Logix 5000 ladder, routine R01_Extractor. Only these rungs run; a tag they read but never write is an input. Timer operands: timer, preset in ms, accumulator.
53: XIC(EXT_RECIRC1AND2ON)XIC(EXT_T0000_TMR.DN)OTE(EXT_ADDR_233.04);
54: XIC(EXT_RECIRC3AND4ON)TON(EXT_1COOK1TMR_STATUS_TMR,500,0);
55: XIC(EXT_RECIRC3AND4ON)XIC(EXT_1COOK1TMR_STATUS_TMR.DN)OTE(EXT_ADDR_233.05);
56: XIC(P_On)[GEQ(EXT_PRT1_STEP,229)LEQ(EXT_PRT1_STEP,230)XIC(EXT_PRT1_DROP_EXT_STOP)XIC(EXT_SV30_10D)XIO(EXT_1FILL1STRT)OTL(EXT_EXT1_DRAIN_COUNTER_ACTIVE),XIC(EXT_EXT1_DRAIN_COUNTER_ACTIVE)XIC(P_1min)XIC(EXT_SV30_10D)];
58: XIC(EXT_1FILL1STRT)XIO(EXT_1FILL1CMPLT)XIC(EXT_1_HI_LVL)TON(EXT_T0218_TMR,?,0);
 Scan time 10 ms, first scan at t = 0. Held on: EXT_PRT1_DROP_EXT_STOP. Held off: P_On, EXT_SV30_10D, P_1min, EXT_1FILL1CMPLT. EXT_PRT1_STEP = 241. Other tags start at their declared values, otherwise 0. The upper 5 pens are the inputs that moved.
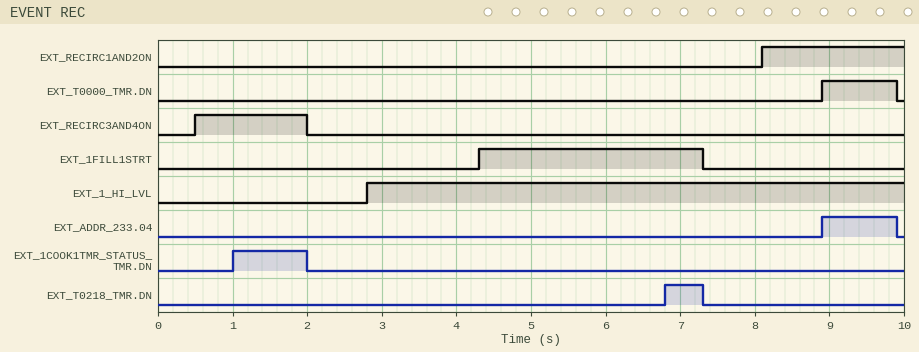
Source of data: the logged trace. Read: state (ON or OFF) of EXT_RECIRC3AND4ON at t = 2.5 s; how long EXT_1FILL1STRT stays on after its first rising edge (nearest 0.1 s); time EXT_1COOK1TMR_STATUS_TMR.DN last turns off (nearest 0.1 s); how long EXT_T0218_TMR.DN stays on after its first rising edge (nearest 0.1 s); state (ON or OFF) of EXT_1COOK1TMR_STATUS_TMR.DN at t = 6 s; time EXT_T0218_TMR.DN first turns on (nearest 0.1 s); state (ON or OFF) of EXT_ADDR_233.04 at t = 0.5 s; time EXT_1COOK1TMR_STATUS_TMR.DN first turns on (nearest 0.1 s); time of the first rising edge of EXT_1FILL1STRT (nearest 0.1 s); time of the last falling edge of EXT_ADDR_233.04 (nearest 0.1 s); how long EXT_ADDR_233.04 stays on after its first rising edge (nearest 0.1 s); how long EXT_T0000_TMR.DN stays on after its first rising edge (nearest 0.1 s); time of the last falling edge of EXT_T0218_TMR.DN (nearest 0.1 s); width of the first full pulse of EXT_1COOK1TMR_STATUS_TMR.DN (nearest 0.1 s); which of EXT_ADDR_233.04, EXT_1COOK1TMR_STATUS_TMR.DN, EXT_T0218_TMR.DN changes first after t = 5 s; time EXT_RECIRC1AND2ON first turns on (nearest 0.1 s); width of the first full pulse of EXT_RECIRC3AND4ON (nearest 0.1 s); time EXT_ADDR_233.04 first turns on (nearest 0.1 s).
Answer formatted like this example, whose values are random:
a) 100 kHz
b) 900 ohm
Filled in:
a) OFF
b) 3.0 s
c) 2.0 s
d) 0.5 s
e) OFF
f) 6.8 s
g) OFF
h) 1.0 s
i) 4.3 s
j) 9.9 s
k) 1.0 s
l) 1.0 s
m) 7.3 s
n) 1.0 s
o) EXT_T0218_TMR.DN
p) 8.1 s
q) 1.5 s
r) 8.9 s
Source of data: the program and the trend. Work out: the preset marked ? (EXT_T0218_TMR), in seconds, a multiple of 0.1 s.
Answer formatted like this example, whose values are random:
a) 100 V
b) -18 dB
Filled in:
a) 2.5 s
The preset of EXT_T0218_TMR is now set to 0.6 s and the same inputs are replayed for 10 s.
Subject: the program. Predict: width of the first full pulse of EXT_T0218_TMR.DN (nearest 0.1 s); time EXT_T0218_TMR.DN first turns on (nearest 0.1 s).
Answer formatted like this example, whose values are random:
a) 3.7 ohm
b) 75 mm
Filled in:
a) 2.4 s
b) 4.9 s
